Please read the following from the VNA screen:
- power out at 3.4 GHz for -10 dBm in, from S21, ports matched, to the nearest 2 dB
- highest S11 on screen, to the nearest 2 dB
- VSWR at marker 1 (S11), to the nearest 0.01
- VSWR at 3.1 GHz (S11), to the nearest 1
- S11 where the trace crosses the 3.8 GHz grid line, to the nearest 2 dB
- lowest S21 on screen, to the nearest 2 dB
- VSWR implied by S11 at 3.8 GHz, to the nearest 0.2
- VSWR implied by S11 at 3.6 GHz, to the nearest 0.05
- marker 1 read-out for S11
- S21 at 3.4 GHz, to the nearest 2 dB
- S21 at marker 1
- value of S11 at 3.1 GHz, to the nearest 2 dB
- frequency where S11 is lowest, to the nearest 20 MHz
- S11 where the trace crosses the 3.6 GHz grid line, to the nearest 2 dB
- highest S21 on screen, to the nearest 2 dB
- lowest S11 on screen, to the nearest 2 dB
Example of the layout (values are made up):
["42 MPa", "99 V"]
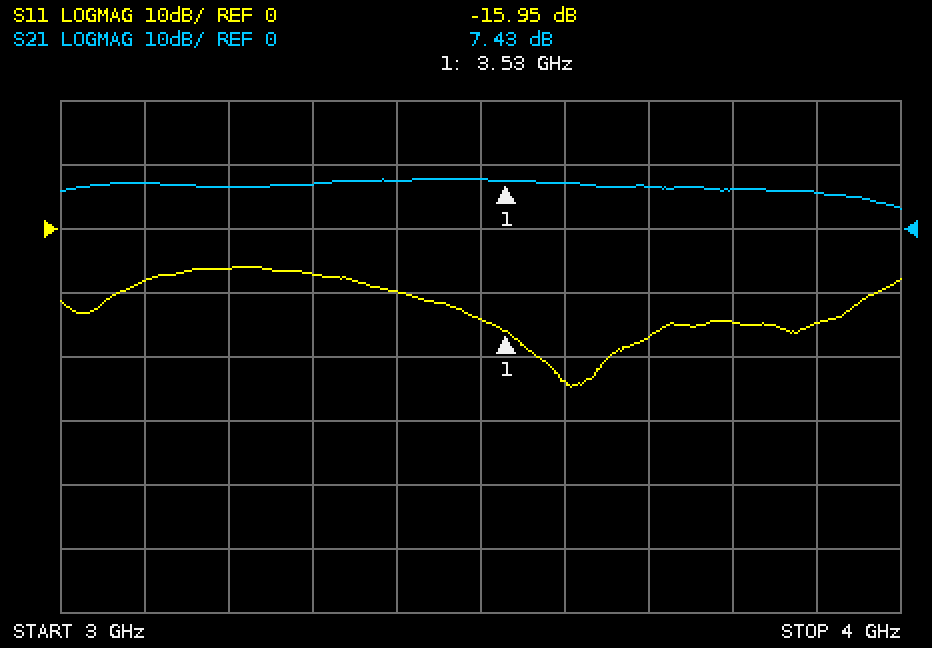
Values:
["-2 dBm", "-6 dB", "1.38", "2", "-14 dB", "4 dB", "1.4", "1.15", "-15.95 dB", "8 dB", "7.43 dB", "-8 dB", "3.60 GHz", "-24 dB", "8 dB", "-24 dB"]
